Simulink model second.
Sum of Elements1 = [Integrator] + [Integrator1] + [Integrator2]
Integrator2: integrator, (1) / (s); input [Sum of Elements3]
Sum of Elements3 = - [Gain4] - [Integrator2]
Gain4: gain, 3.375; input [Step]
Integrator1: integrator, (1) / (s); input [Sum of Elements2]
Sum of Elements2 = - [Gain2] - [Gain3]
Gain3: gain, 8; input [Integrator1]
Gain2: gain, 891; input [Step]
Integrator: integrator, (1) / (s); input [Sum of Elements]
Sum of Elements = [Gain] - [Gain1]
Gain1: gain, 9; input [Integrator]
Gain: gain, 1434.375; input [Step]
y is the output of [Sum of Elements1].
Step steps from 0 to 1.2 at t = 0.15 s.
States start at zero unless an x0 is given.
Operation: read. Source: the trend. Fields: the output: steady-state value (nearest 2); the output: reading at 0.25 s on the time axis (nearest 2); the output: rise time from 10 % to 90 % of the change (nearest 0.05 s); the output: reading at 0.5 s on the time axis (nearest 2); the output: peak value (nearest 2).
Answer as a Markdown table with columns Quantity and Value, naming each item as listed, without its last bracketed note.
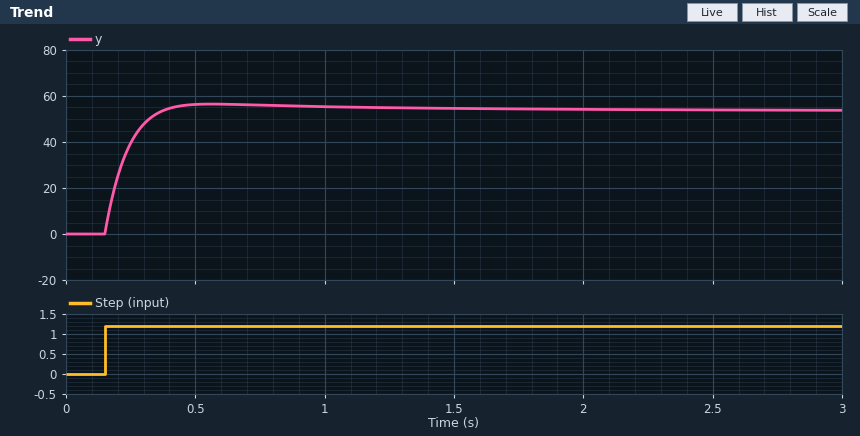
| Quantity | Value |
|---|---|
| the output: steady-state value | 54 |
| the output: reading at 0.25 s on the time axis | 40 |
| the output: rise time from 10 % to 90 % of the change | 0.15 s |
| the output: reading at 0.5 s on the time axis | 56 |
| the output: peak value | 56 |
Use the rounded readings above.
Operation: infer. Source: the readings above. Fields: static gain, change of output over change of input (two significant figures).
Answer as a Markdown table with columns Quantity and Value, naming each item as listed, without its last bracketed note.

| Quantity | Value |
|---|---|
| static gain, change of output over change of input | 45 |
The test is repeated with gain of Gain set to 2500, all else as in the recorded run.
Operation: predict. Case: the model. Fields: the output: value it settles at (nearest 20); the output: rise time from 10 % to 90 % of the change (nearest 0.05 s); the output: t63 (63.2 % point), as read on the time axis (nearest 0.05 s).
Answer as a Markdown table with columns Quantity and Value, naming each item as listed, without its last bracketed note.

| Quantity | Value |
|---|---|
| the output: value it settles at | 200 |
| the output: rise time from 10 % to 90 % of the change | 0.20 s |
| the output: t63 (63.2 % point), as read on the time axis | 0.25 s |
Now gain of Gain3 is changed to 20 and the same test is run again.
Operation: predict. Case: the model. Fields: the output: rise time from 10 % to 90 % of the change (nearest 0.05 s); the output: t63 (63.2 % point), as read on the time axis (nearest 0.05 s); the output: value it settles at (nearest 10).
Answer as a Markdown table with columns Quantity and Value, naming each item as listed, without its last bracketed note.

| Quantity | Value |
|---|---|
| the output: rise time from 10 % to 90 % of the change | 0.25 s |
| the output: t63 (63.2 % point), as read on the time axis | 0.30 s |
| the output: value it settles at | 130 |
